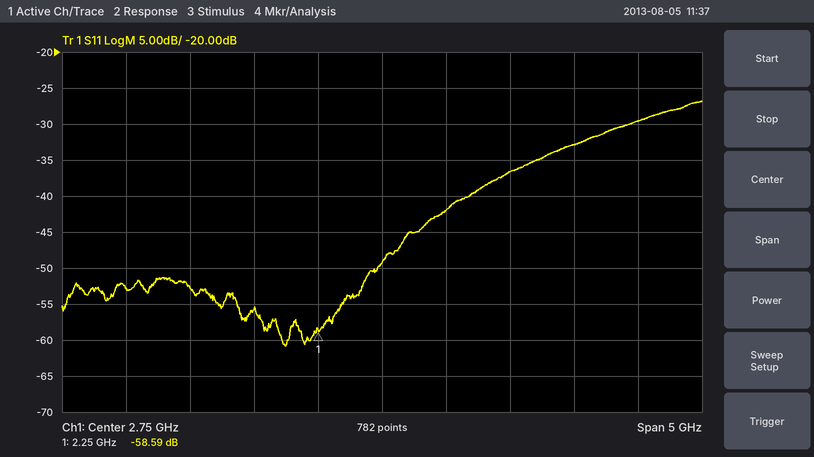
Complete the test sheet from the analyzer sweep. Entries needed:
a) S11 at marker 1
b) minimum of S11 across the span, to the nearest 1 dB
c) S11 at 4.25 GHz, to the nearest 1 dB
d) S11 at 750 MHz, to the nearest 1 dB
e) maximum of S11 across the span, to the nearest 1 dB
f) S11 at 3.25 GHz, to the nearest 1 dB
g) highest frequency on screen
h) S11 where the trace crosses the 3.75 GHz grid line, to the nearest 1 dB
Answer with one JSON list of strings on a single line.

["-58.59 dB", "-61 dB", "-33 dB", "-53 dB", "-27 dB", "-42 dB", "5.25 GHz", "-37 dB"]
